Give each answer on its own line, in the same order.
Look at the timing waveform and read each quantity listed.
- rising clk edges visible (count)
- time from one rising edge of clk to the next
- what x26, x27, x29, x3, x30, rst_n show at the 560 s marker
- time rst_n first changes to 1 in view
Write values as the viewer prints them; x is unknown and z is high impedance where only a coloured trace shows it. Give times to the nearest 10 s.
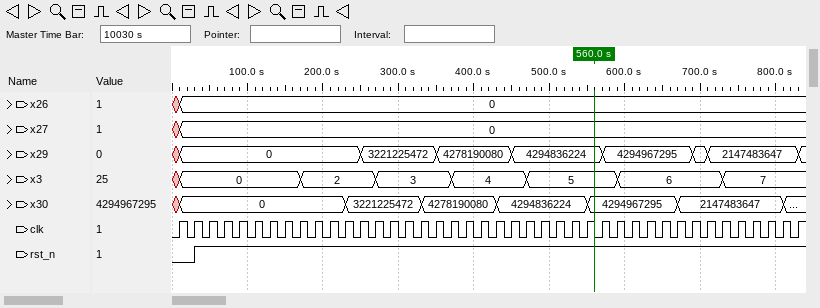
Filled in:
42
20 s
x26=0, x27=0, x29=4294836224, x3=5, x30=4294967295, rst_n=1
30 s
